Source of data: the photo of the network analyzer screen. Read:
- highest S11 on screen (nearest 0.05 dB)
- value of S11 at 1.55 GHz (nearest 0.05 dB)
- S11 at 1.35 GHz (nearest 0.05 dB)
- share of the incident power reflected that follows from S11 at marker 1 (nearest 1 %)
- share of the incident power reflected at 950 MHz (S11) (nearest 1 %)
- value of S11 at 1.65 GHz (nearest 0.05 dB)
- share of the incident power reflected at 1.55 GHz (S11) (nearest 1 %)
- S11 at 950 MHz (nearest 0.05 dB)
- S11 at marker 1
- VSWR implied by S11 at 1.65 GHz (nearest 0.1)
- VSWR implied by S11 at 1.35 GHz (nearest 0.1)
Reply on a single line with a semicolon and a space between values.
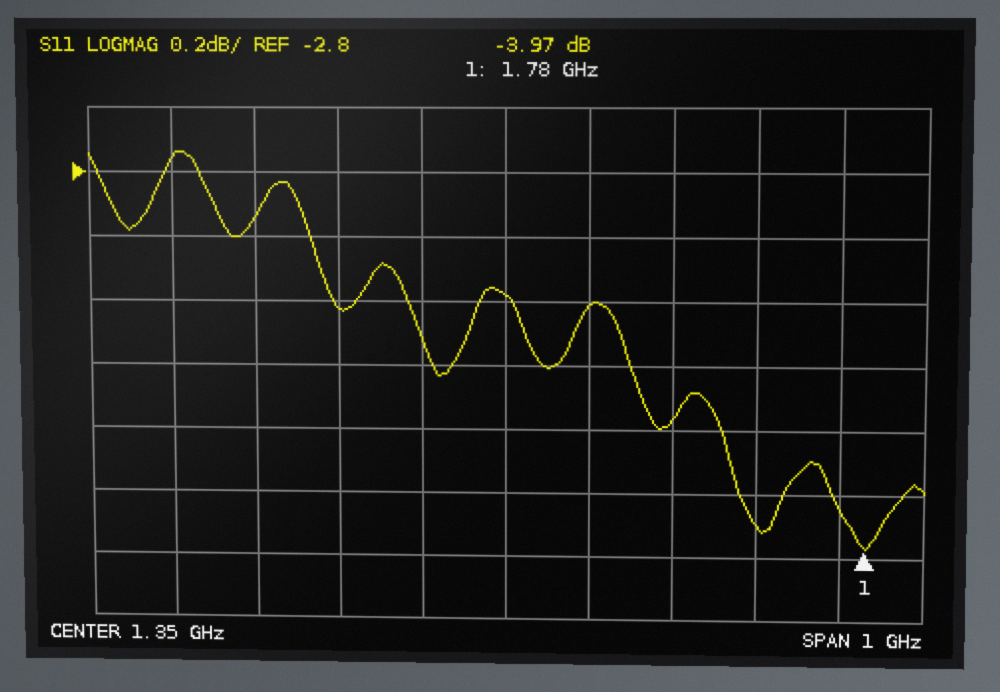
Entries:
-2.75 dB; -3.55 dB; -3.20 dB; 40 %; 53 %; -3.90 dB; 44 %; -2.75 dB; -3.97 dB; 4.5; 5.5
